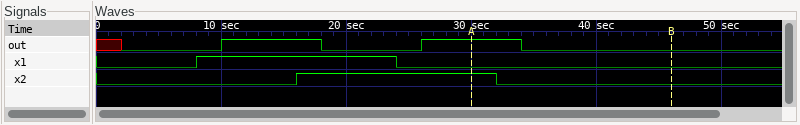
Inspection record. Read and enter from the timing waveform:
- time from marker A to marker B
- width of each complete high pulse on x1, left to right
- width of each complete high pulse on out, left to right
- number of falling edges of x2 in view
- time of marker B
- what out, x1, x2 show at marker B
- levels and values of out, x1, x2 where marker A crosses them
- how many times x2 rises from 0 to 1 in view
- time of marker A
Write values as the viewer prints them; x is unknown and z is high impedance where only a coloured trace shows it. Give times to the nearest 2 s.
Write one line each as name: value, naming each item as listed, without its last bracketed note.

time from marker A to marker B: 16 s
width of each complete high pulse on x1, left to right: 16 s
width of each complete high pulse on out, left to right: 8 s, 8 s
number of falling edges of x2 in view: 1
time of marker B: 46 s
what out, x1, x2 show at marker B: out=0, x1=0, x2=0
levels and values of out, x1, x2 where marker A crosses them: out=1, x1=0, x2=1
how many times x2 rises from 0 to 1 in view: 1
time of marker A: 30 s
